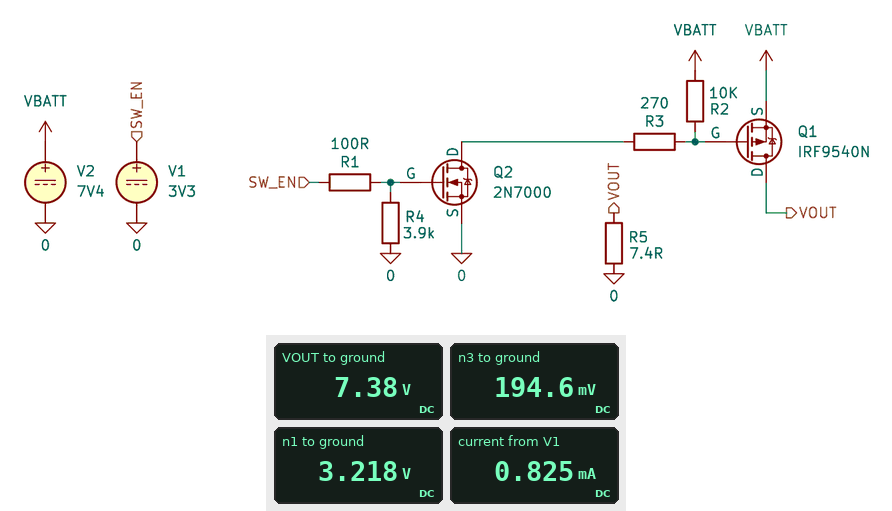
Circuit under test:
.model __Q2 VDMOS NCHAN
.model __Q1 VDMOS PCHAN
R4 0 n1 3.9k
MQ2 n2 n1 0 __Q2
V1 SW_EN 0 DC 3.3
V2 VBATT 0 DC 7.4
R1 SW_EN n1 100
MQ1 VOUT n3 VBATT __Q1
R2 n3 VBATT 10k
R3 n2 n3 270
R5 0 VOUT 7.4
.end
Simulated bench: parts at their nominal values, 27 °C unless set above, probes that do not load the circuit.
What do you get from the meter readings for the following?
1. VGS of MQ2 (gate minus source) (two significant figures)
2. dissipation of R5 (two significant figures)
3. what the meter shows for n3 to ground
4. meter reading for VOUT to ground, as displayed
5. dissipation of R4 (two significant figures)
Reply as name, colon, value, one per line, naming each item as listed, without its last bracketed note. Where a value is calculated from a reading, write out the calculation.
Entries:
VGS of MQ2 (gate minus source): 3.218 V = 3.2 V
dissipation of R5: (7.38 V)^2 / 7.4 Ω = 7.4 W
what the meter shows for n3 to ground: 194.6 mV
meter reading for VOUT to ground, as displayed: 7.38 V
dissipation of R4: (3.218 V)^2 / 3.9 kΩ = 2.7 mW
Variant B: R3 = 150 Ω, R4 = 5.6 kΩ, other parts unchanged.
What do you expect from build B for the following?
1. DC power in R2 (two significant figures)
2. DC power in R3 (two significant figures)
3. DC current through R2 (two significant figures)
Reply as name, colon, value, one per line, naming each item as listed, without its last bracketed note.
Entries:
DC power in R2: 5.3 mW
DC power in R3: 80 µW
DC current through R2: 730 µA
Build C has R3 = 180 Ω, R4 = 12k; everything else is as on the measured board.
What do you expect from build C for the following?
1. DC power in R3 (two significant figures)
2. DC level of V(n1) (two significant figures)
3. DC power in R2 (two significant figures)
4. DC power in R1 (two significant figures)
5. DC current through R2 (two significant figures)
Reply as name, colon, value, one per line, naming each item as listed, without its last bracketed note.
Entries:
DC power in R3: 95 µW
DC level of V(n1): 3.3 V
DC power in R2: 5.3 mW
DC power in R1: 7.4 µW
DC current through R2: 730 µA
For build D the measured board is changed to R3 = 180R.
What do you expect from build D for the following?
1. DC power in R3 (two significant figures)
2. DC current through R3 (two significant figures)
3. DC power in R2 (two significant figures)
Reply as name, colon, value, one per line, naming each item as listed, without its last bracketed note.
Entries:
DC power in R3: 95 µW
DC current through R3: 730 µA
DC power in R2: 5.3 mW
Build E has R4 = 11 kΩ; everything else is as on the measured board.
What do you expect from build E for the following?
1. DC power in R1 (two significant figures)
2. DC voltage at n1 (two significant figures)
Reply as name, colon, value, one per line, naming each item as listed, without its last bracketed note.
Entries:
DC power in R1: 8.8 µW
DC voltage at n1: 3.3 V
